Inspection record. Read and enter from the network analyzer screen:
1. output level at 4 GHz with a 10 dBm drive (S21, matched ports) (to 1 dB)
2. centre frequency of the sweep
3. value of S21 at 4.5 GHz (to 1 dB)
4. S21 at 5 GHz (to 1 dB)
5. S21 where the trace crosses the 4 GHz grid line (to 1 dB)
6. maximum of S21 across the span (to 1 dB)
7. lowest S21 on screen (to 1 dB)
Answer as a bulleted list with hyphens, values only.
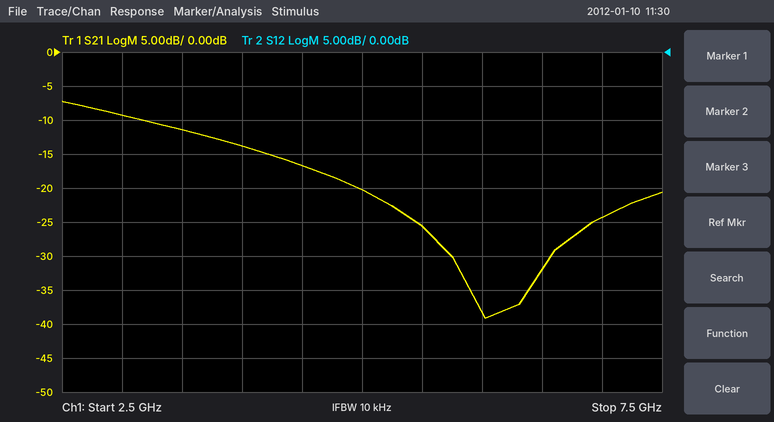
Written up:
- -4 dBm
- 5 GHz
- -17 dB
- -20 dB
- -14 dB
- -7 dB
- -39 dB
